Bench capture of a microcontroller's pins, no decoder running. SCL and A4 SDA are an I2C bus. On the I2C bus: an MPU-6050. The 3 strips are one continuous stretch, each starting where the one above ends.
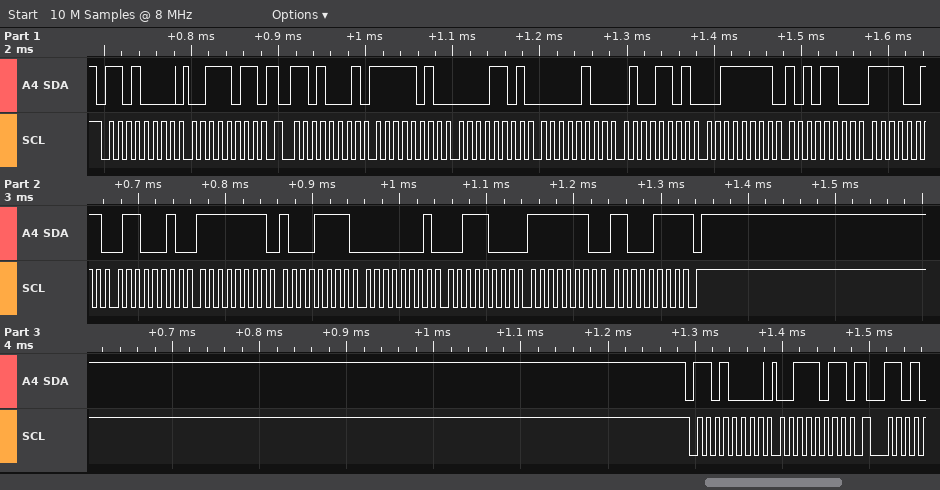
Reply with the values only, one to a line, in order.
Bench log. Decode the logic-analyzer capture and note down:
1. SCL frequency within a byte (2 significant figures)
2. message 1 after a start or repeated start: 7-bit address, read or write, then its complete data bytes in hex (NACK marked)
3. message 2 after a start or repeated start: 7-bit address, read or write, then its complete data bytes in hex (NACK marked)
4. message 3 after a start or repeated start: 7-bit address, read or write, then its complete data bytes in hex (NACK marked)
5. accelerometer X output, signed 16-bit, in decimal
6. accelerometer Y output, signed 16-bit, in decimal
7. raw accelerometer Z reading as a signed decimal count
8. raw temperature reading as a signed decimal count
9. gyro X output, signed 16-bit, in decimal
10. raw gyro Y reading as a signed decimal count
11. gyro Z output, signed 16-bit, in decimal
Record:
100 kHz
0x68 write: 3B
0x68 read: FA 0D 04 4D 3F AC F3 62 FF 8F 01 38 FE C7 NACK
0x68 write: 3B
-1523
1101
16300
-3230
-113
312
-313
